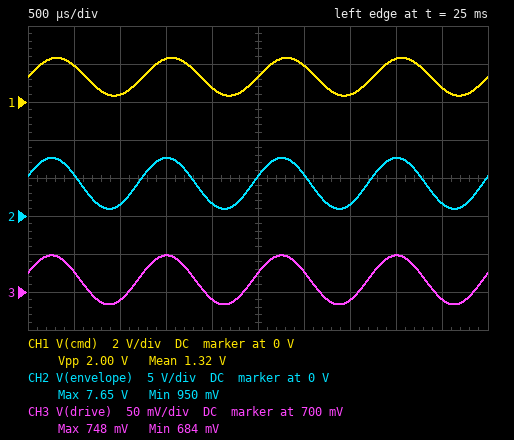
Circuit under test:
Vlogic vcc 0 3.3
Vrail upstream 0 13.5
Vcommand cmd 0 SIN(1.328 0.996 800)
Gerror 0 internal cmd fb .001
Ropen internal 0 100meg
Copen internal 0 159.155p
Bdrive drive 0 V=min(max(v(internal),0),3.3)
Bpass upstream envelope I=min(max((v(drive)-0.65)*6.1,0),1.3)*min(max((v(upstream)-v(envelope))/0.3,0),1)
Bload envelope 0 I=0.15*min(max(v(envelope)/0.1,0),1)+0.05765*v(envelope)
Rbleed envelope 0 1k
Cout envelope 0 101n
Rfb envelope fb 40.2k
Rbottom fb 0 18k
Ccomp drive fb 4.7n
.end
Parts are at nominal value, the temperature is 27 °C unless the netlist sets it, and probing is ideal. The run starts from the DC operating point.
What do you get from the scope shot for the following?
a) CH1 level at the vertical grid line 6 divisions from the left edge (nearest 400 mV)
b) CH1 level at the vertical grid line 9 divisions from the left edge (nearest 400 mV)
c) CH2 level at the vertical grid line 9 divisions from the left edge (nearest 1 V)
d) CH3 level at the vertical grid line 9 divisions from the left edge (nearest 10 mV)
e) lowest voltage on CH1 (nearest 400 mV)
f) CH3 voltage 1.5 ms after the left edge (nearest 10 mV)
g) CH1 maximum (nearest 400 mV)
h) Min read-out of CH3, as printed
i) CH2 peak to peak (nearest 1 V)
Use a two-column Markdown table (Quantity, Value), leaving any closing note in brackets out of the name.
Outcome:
| Quantity | Value |
|---|---|
| CH1 level at the vertical grid line 6 divisions from the left edge | 2.0 V |
| CH1 level at the vertical grid line 9 divisions from the left edge | 800 mV |
| CH2 level at the vertical grid line 9 divisions from the left edge | 2 V |
| CH3 level at the vertical grid line 9 divisions from the left edge | 690 mV |
| lowest voltage on CH1 | 400 mV |
| CH3 voltage 1.5 ms after the left edge | 750 mV |
| CH1 maximum | 2.4 V |
| Min read-out of CH3, as printed | 684 mV |
| CH2 peak to peak | 7 V |
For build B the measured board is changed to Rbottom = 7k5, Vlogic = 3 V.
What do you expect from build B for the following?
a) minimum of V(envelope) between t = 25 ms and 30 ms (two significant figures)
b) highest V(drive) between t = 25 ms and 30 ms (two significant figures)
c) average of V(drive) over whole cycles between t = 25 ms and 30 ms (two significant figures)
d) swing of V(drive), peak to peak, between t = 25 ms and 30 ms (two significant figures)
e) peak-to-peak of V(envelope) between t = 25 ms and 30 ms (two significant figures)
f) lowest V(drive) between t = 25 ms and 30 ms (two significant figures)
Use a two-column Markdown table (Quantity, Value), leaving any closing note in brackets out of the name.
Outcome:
| Quantity | Value |
|---|---|
| minimum of V(envelope) between t = 25 ms and 30 ms | 2.0 V |
| highest V(drive) between t = 25 ms and 30 ms | 2.4 V |
| average of V(drive) over whole cycles between t = 25 ms and 30 ms | 1.1 V |
| swing of V(drive), peak to peak, between t = 25 ms and 30 ms | 1.7 V |
| peak-to-peak of V(envelope) between t = 25 ms and 30 ms | 11 V |
| lowest V(drive) between t = 25 ms and 30 ms | 690 mV |
